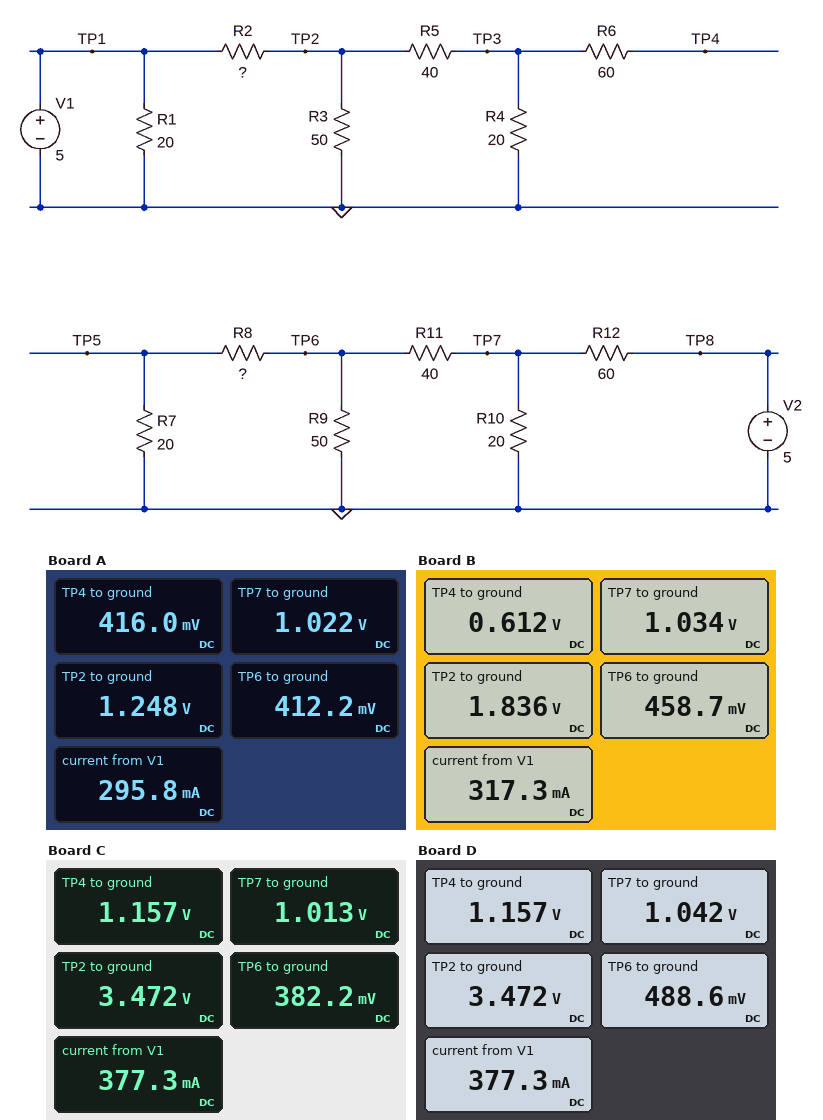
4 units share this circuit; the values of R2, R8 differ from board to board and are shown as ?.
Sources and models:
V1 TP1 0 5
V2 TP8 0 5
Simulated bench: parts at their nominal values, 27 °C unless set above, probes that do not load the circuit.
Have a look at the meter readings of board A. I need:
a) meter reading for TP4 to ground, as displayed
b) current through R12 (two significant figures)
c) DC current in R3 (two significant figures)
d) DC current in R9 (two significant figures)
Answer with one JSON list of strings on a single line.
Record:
["416.0 mV", "66 mA", "25 mA", "8.2 mA"]
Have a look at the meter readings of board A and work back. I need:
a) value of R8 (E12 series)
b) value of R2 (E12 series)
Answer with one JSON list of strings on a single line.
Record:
["39 Ω", "82 Ω"]
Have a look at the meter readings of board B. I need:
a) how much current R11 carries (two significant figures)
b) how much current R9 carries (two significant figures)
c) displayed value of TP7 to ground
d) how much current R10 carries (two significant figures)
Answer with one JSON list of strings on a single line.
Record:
["14 mA", "9.2 mA", "1.034 V", "52 mA"]
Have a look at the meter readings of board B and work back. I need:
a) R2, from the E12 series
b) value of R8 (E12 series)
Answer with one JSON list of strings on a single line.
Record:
["47 Ω", "68 Ω"]
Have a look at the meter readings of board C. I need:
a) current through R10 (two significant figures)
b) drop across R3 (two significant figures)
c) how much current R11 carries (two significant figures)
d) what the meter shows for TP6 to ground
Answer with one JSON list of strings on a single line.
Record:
["51 mA", "3.5 V", "16 mA", "382.2 mV"]
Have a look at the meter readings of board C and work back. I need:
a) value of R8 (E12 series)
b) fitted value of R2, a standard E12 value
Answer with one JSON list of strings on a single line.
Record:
["27 Ω", "12 Ω"]
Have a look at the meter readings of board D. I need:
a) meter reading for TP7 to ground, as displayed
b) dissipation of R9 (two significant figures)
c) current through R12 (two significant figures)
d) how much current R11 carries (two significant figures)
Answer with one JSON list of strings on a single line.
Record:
["1.042 V", "4.8 mW", "66 mA", "14 mA"]
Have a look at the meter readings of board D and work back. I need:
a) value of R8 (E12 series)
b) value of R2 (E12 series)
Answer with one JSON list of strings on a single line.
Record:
["100 Ω", "12 Ω"]
